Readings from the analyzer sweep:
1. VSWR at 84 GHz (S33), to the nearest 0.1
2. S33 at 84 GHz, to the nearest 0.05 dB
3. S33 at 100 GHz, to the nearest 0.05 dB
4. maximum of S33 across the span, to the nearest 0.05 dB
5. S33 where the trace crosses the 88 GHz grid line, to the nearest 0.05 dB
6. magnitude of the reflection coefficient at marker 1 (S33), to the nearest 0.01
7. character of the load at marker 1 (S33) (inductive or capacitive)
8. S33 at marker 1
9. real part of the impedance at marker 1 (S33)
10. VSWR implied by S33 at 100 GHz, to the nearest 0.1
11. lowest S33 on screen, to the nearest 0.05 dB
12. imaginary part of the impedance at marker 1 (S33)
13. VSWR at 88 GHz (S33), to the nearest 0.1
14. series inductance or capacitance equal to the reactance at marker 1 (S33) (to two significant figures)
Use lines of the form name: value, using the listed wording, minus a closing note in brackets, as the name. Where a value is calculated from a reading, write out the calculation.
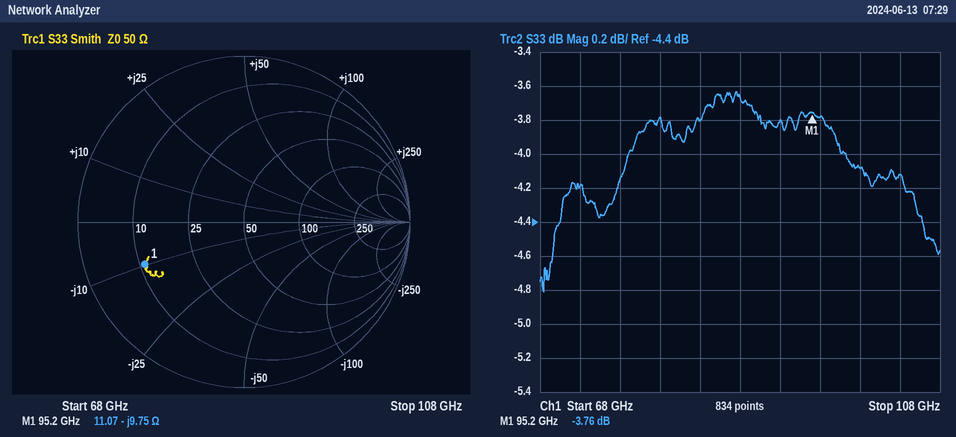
VSWR at 84 GHz (S33), to the nearest 0.1: |Γ| = 10^(-3.8/20) = 0.6457; VSWR = (1 + 0.6457)/(1 − 0.6457) ≈ 4.6
S33 at 84 GHz, to the nearest 0.05 dB: -3.80 dB
S33 at 100 GHz, to the nearest 0.05 dB: -4.10 dB
maximum of S33 across the span, to the nearest 0.05 dB: -3.65 dB
S33 where the trace crosses the 88 GHz grid line, to the nearest 0.05 dB: -3.65 dB
magnitude of the reflection coefficient at marker 1 (S33), to the nearest 0.01: 0.65
character of the load at marker 1 (S33): capacitive
S33 at marker 1: -3.76 dB
real part of the impedance at marker 1: 11.07 Ω
VSWR implied by S33 at 100 GHz, to the nearest 0.1: |Γ| = 10^(-4.1/20) = 0.6237; VSWR = (1 + 0.6237)/(1 − 0.6237) ≈ 4.3
lowest S33 on screen, to the nearest 0.05 dB: -4.80 dB
imaginary part of the impedance at marker 1: -9.75 Ω
VSWR at 88 GHz (S33), to the nearest 0.1: |Γ| = 10^(-3.65/20) = 0.6569; VSWR = (1 + 0.6569)/(1 − 0.6569) ≈ 4.8
series inductance or capacitance equal to the reactance at marker 1 (S33): C = 1/(2π × 95.2 GHz × 9.75 Ω) ≈ 171 fF, so 170 fF to two significant figures
